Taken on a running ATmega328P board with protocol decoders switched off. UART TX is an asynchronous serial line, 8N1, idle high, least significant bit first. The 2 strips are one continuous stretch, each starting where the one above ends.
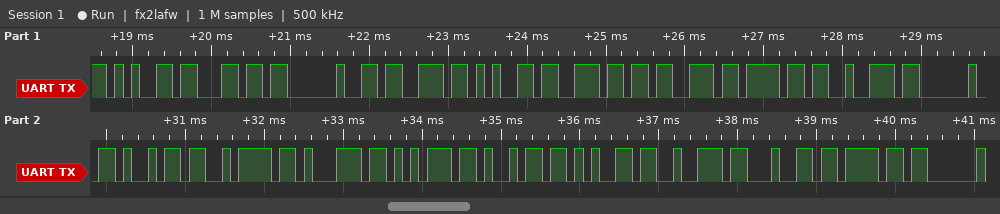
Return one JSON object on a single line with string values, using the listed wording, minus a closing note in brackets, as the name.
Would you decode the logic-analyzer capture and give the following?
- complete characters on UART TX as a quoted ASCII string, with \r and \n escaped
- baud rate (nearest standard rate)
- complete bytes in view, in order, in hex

{"complete characters on UART TX as a quoted ASCII string, with \\r and \\n escaped": "\"el sensor izquierdo\"", "baud rate": "9600 baud", "complete bytes in view, in order, in hex": "0x65 0x6C 0x20 0x73 0x65 0x6E 0x73 0x6F 0x72 0x20 0x69 0x7A 0x71 0x75 0x69 0x65 0x72 0x64 0x6F"}
